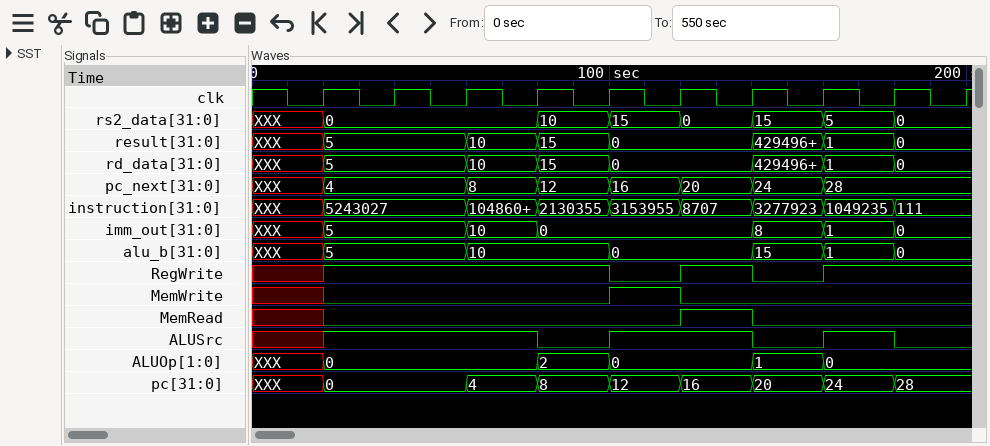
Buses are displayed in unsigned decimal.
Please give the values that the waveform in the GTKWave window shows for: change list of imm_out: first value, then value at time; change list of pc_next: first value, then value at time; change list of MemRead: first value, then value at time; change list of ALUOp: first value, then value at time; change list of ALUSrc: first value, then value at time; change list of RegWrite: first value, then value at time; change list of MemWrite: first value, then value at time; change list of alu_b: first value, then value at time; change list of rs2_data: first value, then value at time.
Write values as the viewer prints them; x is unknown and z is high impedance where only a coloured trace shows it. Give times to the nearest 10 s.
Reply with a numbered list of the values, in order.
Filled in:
1. XXX, 5 at 20 s, 10 at 60 s, 0 at 80 s, 8 at 140 s, 1 at 160 s, 0 at 180 s
2. XXX, 4 at 20 s, 8 at 60 s, 12 at 80 s, 16 at 100 s, 20 at 120 s, 24 at 140 s, 28 at 160 s
3. x, 0 at 20 s, 1 at 120 s, 0 at 140 s
4. XXX, 0 at 20 s, 2 at 80 s, 0 at 100 s, 1 at 140 s, 0 at 160 s
5. x, 1 at 20 s, 0 at 80 s, 1 at 100 s, 0 at 140 s, 1 at 160 s, 0 at 180 s
6. x, 1 at 20 s, 0 at 100 s, 1 at 120 s, 0 at 140 s, 1 at 160 s
7. x, 0 at 20 s, 1 at 100 s, 0 at 120 s
8. XXX, 5 at 20 s, 10 at 60 s, 0 at 100 s, 15 at 140 s, 1 at 160 s, 0 at 180 s
9. XXX, 0 at 20 s, 10 at 80 s, 15 at 100 s, 0 at 120 s, 15 at 140 s, 5 at 160 s, 0 at 180 s
